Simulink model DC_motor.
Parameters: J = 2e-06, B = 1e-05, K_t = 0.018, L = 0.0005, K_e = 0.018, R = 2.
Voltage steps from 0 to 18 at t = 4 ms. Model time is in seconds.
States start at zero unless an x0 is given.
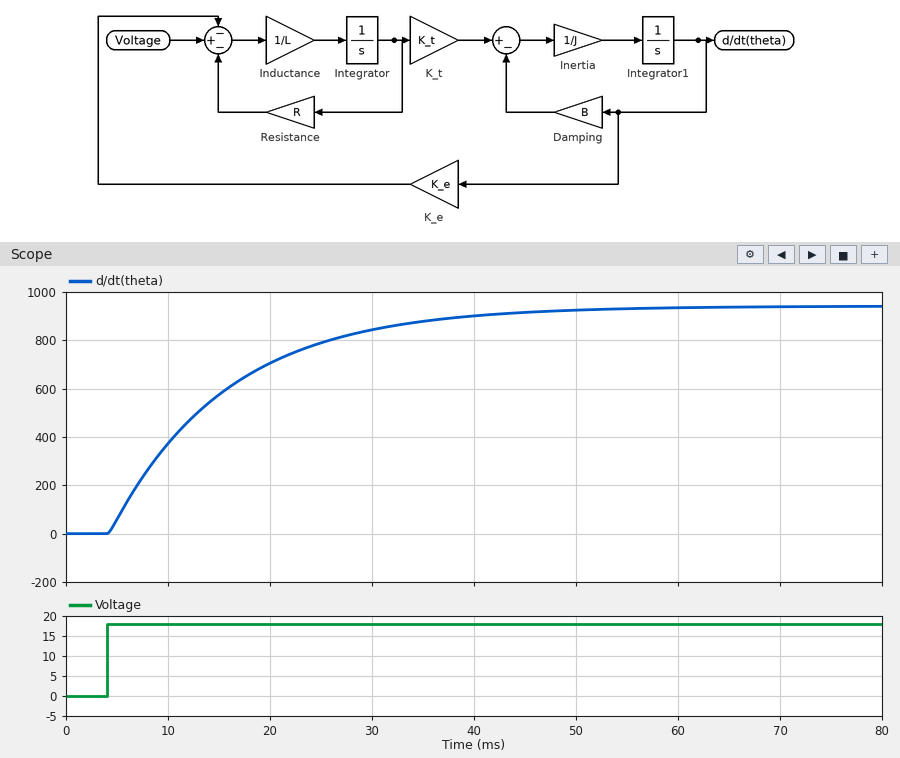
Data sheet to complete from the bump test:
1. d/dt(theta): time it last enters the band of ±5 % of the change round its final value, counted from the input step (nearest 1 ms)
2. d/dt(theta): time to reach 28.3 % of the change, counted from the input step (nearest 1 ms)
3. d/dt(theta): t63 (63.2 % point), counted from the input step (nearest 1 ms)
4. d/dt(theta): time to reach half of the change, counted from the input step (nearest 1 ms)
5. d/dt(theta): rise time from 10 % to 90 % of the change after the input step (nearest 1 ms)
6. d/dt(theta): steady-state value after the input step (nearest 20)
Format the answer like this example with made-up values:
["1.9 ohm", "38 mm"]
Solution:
["34 ms", "4 ms", "12 ms", "8 ms", "25 ms", "940"]
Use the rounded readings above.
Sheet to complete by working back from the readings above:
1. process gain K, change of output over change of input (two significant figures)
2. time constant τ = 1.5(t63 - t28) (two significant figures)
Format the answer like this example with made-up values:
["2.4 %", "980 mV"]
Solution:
["52", "12 ms"]
